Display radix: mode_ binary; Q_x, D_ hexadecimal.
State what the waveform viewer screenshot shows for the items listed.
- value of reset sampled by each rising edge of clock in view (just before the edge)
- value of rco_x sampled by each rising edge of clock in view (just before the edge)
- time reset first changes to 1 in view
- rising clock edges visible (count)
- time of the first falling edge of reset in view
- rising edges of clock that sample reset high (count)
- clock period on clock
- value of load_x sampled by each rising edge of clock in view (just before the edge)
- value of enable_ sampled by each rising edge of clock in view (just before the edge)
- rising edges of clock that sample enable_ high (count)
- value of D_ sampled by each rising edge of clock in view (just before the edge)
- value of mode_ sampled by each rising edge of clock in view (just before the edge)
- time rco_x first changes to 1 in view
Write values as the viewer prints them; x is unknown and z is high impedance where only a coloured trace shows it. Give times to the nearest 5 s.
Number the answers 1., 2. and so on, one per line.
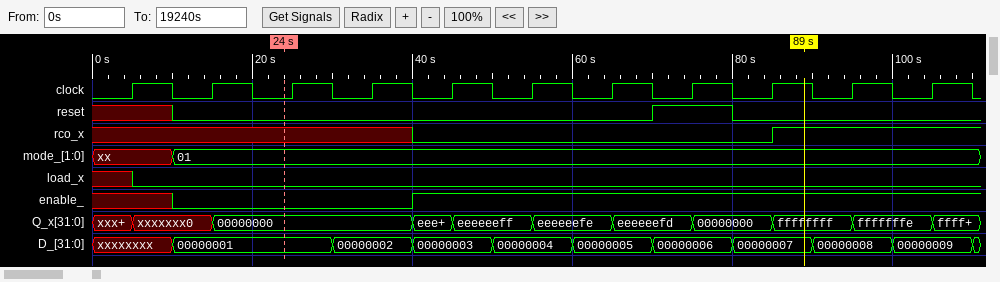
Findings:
1. x 0 0 0 0 0 0 1 0 0 0
2. x x x x 0 0 0 0 0 1 1
3. 70 s
4. 11
5. 80 s
6. 1
7. 10 s
8. x 0 0 0 0 0 0 0 0 0 0
9. x 0 0 0 1 1 1 1 1 1 1
10. 7
11. xxxxxxxx, 00000001, 00000001, 00000002, 00000003, 00000004, 00000005, 00000006, 00000007, 00000008, 00000009
12. xx, 01, 01, 01, 01, 01, 01, 01, 01, 01, 01
13. 85 s
